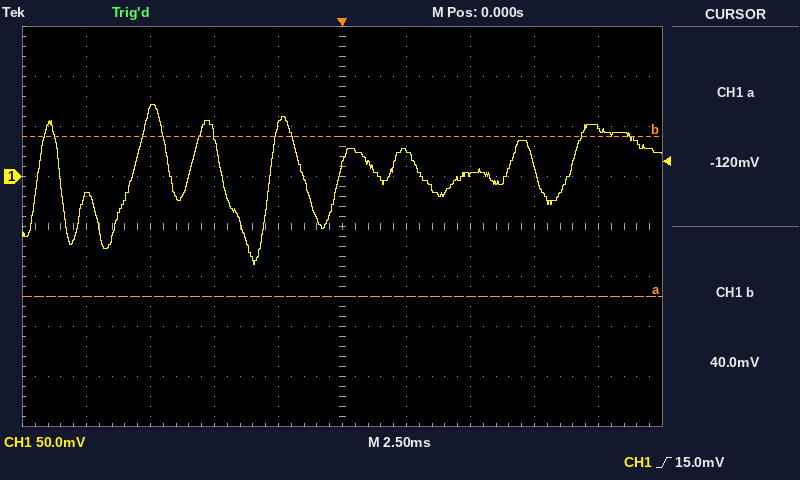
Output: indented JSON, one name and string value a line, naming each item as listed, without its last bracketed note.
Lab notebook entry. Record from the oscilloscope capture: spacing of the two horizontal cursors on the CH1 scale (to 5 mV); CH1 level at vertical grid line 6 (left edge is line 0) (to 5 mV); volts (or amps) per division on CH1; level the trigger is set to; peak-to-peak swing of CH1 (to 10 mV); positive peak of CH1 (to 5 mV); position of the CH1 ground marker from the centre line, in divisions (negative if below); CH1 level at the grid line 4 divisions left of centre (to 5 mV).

{
  "spacing of the two horizontal cursors on the CH1 scale": "160 mV",
  "CH1 level at vertical grid line 6 (left edge is line 0)": "25 mV",
  "volts (or amps) per division on CH1": "50 mV",
  "level the trigger is set to": "15.0 mV",
  "peak-to-peak swing of CH1": "160 mV",
  "positive peak of CH1": "70 mV",
  "position of the CH1 ground marker from the centre line, in divisions": "+1.0 div",
  "CH1 level at the grid line 4 divisions left of centre": "-20 mV"
}
